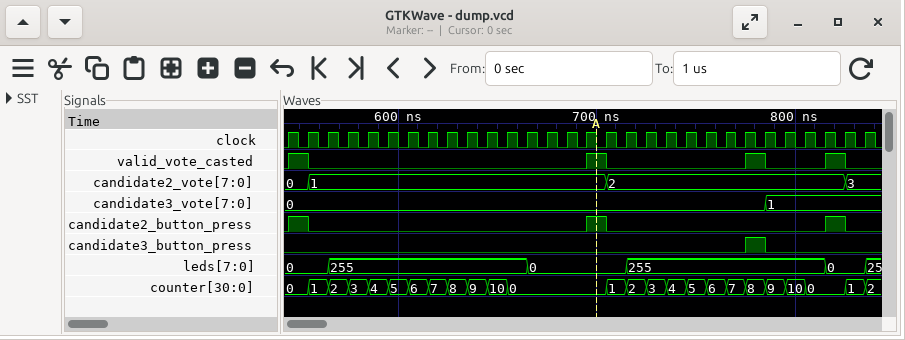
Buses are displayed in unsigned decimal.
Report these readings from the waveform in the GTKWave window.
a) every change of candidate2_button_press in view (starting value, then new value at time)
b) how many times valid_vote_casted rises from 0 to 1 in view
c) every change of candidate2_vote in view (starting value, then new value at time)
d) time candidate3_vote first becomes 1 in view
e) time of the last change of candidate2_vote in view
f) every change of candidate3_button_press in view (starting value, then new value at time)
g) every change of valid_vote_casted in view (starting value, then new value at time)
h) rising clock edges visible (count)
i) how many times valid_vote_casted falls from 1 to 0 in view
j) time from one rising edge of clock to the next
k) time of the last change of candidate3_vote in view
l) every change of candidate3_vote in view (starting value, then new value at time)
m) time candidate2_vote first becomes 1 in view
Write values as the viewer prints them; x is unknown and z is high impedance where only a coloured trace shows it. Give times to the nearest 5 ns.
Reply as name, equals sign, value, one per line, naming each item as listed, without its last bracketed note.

every change of candidate2_button_press in view = 0, 1 at 545 ns, 0 at 555 ns, 1 at 695 ns, 0 at 705 ns, 1 at 815 ns, 0 at 825 ns
how many times valid_vote_casted rises from 0 to 1 in view = 4
every change of candidate2_vote in view = 0, 1 at 555 ns, 2 at 705 ns, 3 at 825 ns
time candidate3_vote first becomes 1 in view = 785 ns
time of the last change of candidate2_vote in view = 825 ns
every change of candidate3_button_press in view = 0, 1 at 775 ns, 0 at 785 ns
every change of valid_vote_casted in view = 0, 1 at 545 ns, 0 at 555 ns, 1 at 695 ns, 0 at 705 ns, 1 at 775 ns, 0 at 785 ns, 1 at 815 ns, 0 at 825 ns
rising clock edges visible = 30
how many times valid_vote_casted falls from 1 to 0 in view = 4
time from one rising edge of clock to the next = 10 ns
time of the last change of candidate3_vote in view = 785 ns
every change of candidate3_vote in view = 0, 1 at 785 ns
time candidate2_vote first becomes 1 in view = 555 ns
